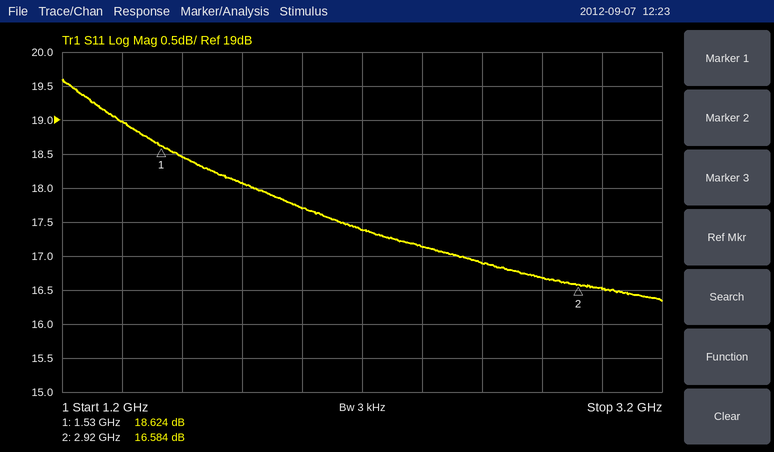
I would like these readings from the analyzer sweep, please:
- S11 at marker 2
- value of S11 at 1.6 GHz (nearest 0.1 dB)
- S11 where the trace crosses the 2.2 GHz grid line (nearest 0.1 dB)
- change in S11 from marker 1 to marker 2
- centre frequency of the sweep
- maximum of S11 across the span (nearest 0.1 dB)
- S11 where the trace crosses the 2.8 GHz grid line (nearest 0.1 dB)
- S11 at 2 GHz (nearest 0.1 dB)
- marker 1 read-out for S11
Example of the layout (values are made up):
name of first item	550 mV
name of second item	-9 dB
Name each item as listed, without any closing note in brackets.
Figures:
S11 at marker 2	16.584 dB
value of S11 at 1.6 GHz	18.5 dB
S11 where the trace crosses the 2.2 GHz grid line	17.4 dB
change in S11 from marker 1 to marker 2	-2.040 dB
centre frequency of the sweep	2.2 GHz
maximum of S11 across the span	19.6 dB
S11 where the trace crosses the 2.8 GHz grid line	16.7 dB
S11 at 2 GHz	17.7 dB
marker 1 read-out for S11	18.624 dB
